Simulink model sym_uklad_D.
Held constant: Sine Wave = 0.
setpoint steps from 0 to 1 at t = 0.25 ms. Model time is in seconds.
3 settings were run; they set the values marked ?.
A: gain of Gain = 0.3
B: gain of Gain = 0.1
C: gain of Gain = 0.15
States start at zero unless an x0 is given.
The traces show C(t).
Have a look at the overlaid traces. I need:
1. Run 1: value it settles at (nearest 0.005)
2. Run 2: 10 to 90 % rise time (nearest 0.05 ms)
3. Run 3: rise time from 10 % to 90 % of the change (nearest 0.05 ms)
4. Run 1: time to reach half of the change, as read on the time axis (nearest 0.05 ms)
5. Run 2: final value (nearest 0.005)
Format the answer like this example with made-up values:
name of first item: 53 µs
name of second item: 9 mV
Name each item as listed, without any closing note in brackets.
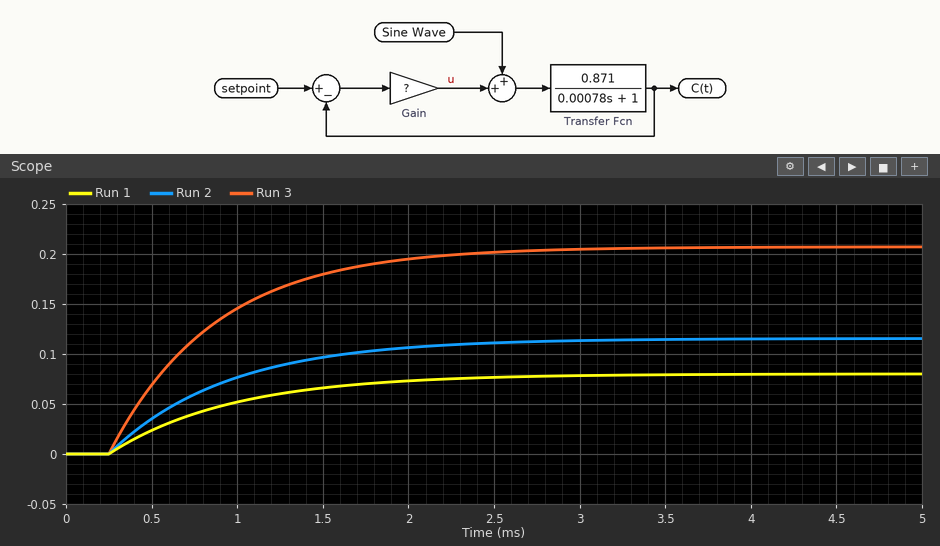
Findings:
Run 1: value it settles at: 0.080
Run 2: 10 to 90 % rise time: 1.50 ms
Run 3: rise time from 10 % to 90 % of the change: 1.35 ms
Run 1: time to reach half of the change, as read on the time axis: 0.75 ms
Run 2: final value: 0.115
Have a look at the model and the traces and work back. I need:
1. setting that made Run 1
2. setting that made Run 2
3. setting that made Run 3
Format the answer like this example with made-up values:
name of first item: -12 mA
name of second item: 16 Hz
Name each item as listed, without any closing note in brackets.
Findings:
setting that made Run 1: B
setting that made Run 2: C
setting that made Run 3: A
